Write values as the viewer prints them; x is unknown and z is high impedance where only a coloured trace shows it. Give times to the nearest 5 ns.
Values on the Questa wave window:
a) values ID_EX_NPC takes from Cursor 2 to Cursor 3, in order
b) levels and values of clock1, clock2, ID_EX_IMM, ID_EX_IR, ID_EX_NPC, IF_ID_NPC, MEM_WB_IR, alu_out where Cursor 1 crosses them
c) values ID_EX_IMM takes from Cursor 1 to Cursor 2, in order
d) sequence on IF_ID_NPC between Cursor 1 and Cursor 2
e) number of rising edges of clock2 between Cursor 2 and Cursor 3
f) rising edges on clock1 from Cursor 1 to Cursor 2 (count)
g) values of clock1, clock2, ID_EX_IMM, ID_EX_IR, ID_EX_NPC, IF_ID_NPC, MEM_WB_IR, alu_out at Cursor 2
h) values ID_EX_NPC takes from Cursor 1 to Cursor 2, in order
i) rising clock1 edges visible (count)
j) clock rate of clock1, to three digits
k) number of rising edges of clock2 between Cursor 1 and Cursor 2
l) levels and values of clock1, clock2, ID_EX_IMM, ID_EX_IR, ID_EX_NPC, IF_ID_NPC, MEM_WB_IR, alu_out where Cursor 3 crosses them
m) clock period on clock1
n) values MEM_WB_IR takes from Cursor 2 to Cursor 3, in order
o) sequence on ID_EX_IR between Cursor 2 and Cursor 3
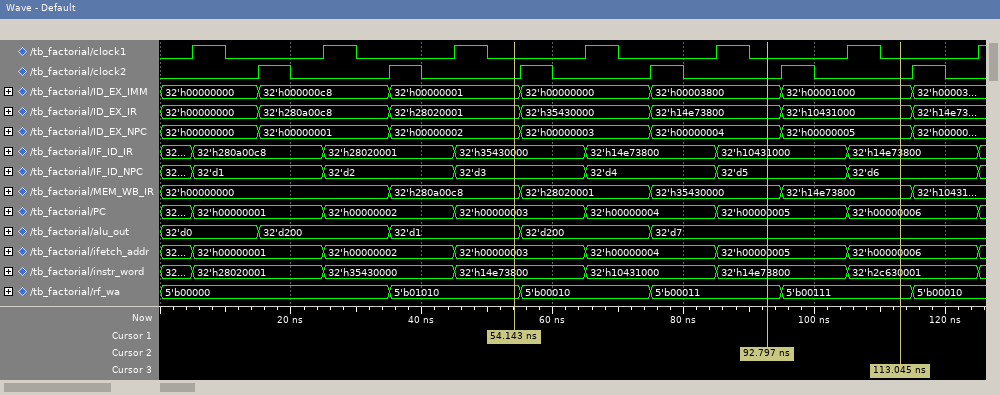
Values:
32'h00000004, 32'h00000005
clock1=0, clock2=0, ID_EX_IMM=32'h00000001, ID_EX_IR=32'h28020001, ID_EX_NPC=32'h00000002, IF_ID_NPC=32'd3, MEM_WB_IR=32'h280a00c8, alu_out=32'd1
32'h00000001, 32'h00000000, 32'h00003800
32'd3, 32'd4, 32'd5
1
2
clock1=0, clock2=0, ID_EX_IMM=32'h00003800, ID_EX_IR=32'h14e73800, ID_EX_NPC=32'h00000004, IF_ID_NPC=32'd5, MEM_WB_IR=32'h35430000, alu_out=32'd7
32'h00000002, 32'h00000003, 32'h00000004
7
50.0 MHz
2
clock1=0, clock2=0, ID_EX_IMM=32'h00001000, ID_EX_IR=32'h10431000, ID_EX_NPC=32'h00000005, IF_ID_NPC=32'd6, MEM_WB_IR=32'h14e73800, alu_out=32'd7
20 ns
32'h35430000, 32'h14e73800
32'h14e73800, 32'h10431000
